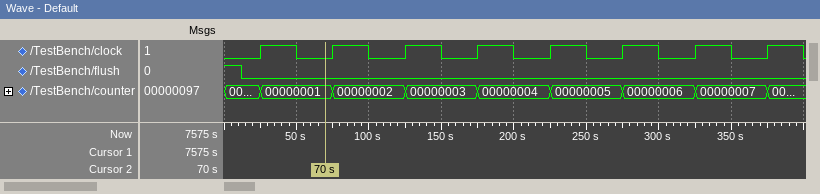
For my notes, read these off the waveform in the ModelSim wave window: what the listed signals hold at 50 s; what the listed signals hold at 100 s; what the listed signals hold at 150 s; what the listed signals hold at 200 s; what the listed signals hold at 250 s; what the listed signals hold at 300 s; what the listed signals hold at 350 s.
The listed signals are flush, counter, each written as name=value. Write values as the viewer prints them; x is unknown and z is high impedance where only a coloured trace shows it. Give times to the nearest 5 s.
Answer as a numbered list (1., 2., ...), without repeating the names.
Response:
1. flush=0, counter=00000001
2. flush=0, counter=00000002
3. flush=0, counter=00000003
4. flush=0, counter=00000004
5. flush=0, counter=00000005
6. flush=0, counter=00000006
7. flush=0, counter=00000007
